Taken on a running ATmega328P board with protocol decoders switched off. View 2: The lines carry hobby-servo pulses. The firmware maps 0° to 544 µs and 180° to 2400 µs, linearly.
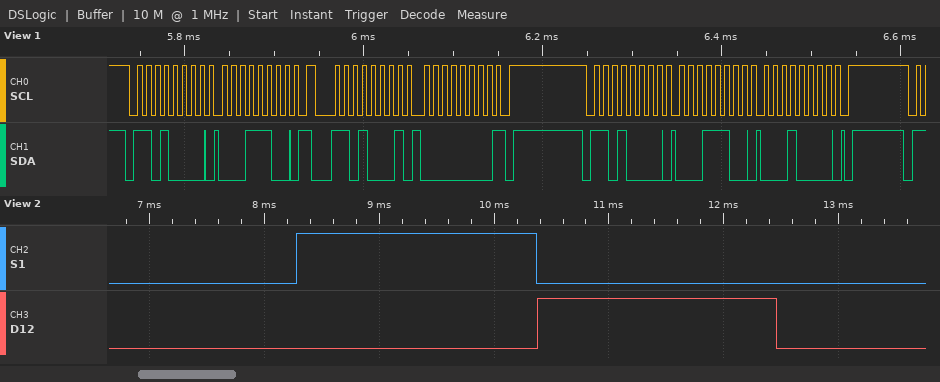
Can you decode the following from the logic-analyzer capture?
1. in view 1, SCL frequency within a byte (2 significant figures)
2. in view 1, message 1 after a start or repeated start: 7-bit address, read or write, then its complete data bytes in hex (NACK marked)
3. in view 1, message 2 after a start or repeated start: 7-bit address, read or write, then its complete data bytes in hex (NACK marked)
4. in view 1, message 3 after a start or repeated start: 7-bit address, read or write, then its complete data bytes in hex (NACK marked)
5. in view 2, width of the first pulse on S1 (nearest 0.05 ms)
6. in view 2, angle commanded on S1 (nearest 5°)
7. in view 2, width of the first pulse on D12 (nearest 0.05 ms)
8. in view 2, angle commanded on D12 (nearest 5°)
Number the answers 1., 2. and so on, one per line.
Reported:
1. 100 kHz
2. 0x68 write: 1C
3. 0x68 read: 00 NACK
4. 0x68 write: 1C 10
5. 2.10 ms
6. 150°
7. 2.10 ms
8. 150°
